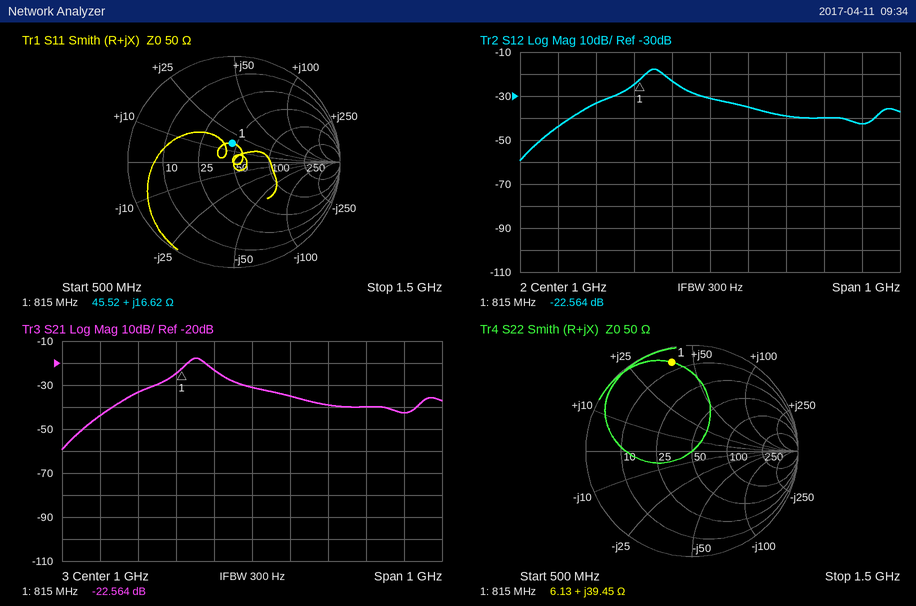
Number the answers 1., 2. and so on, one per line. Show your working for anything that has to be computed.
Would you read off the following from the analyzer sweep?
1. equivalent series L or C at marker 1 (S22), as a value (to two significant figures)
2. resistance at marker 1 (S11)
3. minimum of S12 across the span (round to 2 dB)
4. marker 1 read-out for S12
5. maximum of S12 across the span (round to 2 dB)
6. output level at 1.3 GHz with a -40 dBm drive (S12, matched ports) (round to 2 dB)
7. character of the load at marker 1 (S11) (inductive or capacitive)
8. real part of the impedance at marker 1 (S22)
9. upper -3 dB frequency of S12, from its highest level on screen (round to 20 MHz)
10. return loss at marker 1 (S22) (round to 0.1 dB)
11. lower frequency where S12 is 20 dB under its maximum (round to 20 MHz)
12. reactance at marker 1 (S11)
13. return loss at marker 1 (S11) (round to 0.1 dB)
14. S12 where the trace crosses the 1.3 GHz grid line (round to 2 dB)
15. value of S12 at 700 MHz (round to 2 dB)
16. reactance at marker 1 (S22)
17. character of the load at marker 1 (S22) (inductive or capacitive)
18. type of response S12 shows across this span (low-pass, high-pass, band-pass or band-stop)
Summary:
1. L = 39.45 Ω/(2π × 815 MHz) ≈ 7.7 nH
2. 45.52 Ω
3. -60 dB
4. -22.564 dB
5. -18 dB
6. -40 dBm + (-40 dB) = -80 dBm
7. inductive
8. 6.13 Ω
9. 880 MHz
10. 1.3 dB
11. 660 MHz
12. +16.62 Ω
13. 15.0 dB
14. -40 dB
15. -34 dB
16. +39.45 Ω
17. inductive
18. band-pass
